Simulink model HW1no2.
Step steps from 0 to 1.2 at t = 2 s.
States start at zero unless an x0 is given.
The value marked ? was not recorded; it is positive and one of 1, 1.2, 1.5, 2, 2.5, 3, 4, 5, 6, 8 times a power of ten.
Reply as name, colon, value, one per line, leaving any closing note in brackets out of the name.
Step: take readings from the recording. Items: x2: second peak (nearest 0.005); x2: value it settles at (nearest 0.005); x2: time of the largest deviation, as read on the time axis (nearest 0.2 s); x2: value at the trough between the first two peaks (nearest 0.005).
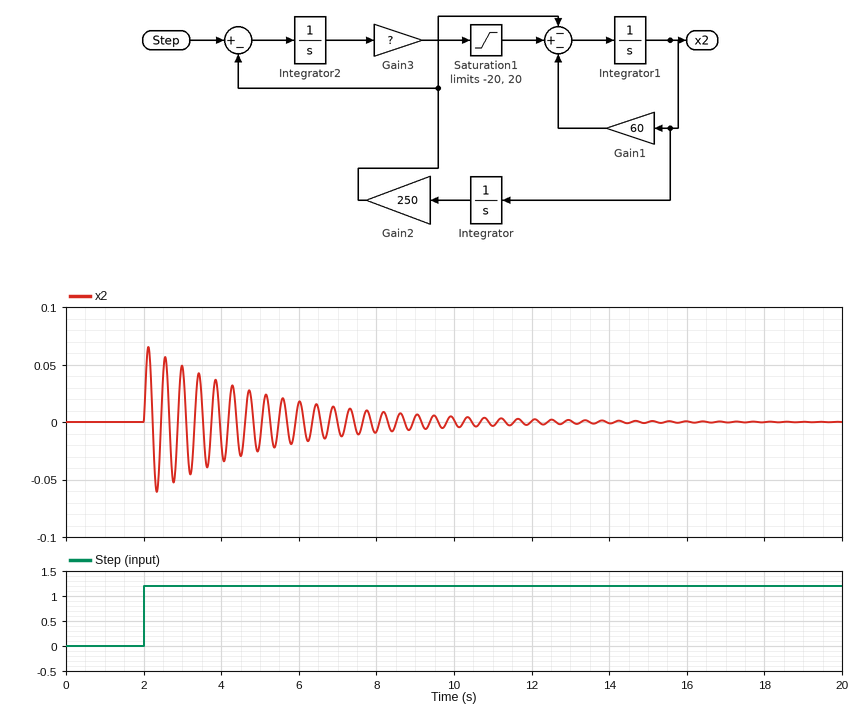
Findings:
x2: second peak: 0.055
x2: value it settles at: 0.000
x2: time of the largest deviation, as read on the time axis: 2.2 s
x2: value at the trough between the first two peaks: -0.060
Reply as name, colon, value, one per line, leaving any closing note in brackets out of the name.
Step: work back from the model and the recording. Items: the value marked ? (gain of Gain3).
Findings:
the value marked ?: 50
